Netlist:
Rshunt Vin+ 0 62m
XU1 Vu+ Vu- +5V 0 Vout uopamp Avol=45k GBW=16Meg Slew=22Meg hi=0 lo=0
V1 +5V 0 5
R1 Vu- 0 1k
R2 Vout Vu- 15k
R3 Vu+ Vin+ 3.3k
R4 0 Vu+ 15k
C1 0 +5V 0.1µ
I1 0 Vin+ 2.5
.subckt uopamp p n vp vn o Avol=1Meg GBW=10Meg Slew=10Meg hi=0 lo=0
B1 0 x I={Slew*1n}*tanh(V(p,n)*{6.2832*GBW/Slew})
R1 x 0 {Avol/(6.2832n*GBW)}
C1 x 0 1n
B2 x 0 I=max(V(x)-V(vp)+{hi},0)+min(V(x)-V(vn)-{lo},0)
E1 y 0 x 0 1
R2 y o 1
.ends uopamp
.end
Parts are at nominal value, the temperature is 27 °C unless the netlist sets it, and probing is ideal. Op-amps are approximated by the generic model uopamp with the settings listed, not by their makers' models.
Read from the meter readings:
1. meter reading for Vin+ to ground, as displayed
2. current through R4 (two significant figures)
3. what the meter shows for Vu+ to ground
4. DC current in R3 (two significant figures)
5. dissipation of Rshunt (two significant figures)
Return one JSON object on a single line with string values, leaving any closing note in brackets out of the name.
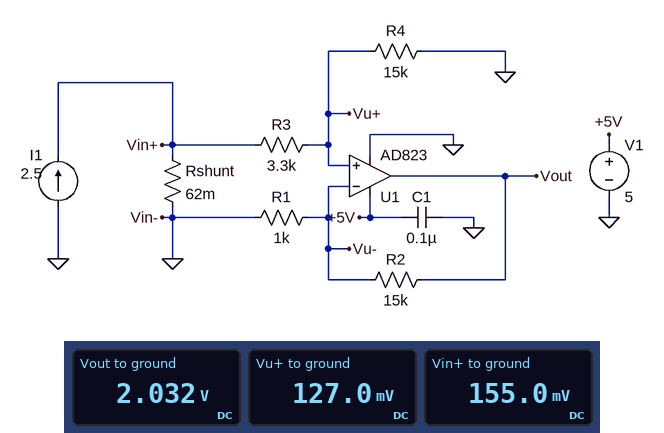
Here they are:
{"meter reading for Vin+ to ground, as displayed": "155.0 mV", "current through R4": "8.5 µA", "what the meter shows for Vu+ to ground": "127.0 mV", "DC current in R3": "8.5 µA", "dissipation of Rshunt": "390 mW"}
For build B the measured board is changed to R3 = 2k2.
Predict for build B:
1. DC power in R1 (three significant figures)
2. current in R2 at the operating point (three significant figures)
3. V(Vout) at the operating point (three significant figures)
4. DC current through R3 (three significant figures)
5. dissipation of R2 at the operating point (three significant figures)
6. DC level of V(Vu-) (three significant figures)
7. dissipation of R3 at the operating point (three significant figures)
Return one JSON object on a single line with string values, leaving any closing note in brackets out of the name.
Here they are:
{"DC power in R1": "18.3 µW", "current in R2 at the operating point": "135 µA", "V(Vout) at the operating point": "2.16 V", "DC current through R3": "9.01 µA", "dissipation of R2 at the operating point": "274 µW", "DC level of V(Vu-)": "135 mV", "dissipation of R3 at the operating point": "179 nW"}
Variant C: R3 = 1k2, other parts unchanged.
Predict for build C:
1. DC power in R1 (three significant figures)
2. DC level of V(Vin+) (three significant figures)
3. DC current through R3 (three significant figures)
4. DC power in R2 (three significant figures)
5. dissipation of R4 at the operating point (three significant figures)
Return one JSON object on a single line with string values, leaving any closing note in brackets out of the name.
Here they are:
{"DC power in R1": "20.6 µW", "DC level of V(Vin+)": "155 mV", "DC current through R3": "9.57 µA", "DC power in R2": "309 µW", "dissipation of R4 at the operating point": "1.37 µW"}
